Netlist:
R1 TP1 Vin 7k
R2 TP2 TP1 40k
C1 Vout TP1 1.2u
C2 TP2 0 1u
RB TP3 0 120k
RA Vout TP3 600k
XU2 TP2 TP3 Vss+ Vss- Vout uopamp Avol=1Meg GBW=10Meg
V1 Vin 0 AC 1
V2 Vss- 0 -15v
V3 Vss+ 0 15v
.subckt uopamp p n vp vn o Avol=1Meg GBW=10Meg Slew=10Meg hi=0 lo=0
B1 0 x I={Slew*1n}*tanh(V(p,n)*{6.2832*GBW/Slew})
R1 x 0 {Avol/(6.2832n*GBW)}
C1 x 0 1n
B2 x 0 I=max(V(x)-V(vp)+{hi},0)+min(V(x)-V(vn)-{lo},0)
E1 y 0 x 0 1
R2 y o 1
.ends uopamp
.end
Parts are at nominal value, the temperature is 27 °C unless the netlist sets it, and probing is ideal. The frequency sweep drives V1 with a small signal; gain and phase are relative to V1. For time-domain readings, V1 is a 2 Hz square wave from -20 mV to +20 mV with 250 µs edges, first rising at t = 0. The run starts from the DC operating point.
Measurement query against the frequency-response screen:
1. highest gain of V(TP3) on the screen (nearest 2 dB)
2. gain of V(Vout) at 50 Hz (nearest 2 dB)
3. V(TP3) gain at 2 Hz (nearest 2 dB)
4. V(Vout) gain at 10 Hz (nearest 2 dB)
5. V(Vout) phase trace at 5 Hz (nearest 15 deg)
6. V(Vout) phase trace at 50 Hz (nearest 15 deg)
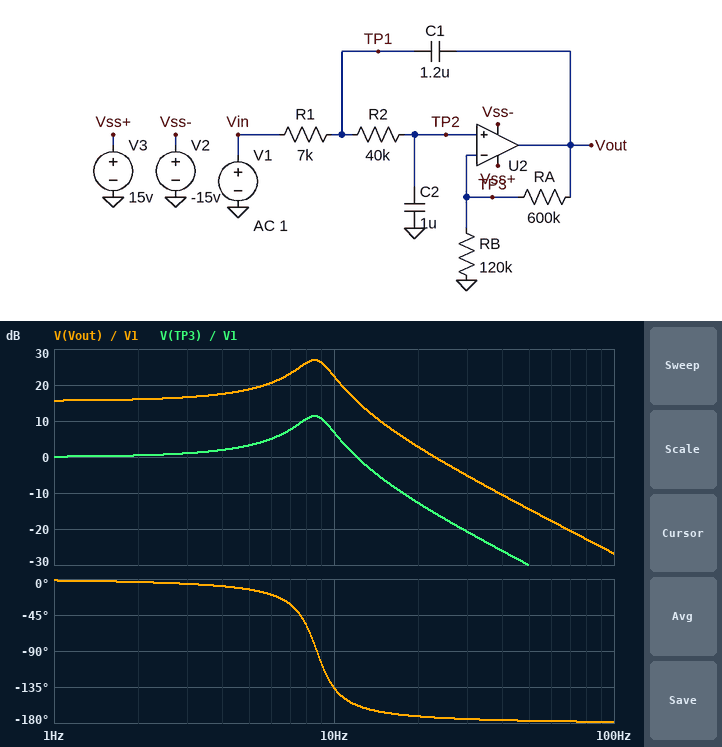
12 dB
-14 dB
0 dB
22 dB
-15 deg
-180 deg
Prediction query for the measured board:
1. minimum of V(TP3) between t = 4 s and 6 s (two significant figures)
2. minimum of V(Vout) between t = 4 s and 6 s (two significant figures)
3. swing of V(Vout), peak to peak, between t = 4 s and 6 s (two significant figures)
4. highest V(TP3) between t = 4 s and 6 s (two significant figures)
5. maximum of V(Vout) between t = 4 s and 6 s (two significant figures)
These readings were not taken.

-43 mV
-260 mV
520 mV
43 mV
260 mV
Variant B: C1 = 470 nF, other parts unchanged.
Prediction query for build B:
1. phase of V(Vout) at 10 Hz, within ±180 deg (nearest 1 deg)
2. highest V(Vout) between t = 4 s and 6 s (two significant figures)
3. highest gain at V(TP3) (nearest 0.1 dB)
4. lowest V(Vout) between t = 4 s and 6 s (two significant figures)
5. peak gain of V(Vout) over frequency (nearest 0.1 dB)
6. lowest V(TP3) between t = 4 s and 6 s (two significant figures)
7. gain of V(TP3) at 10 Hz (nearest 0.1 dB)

-76 deg
120 mV
0 dB
-120 mV
15.6 dB
-20 mV
-5.9 dB
